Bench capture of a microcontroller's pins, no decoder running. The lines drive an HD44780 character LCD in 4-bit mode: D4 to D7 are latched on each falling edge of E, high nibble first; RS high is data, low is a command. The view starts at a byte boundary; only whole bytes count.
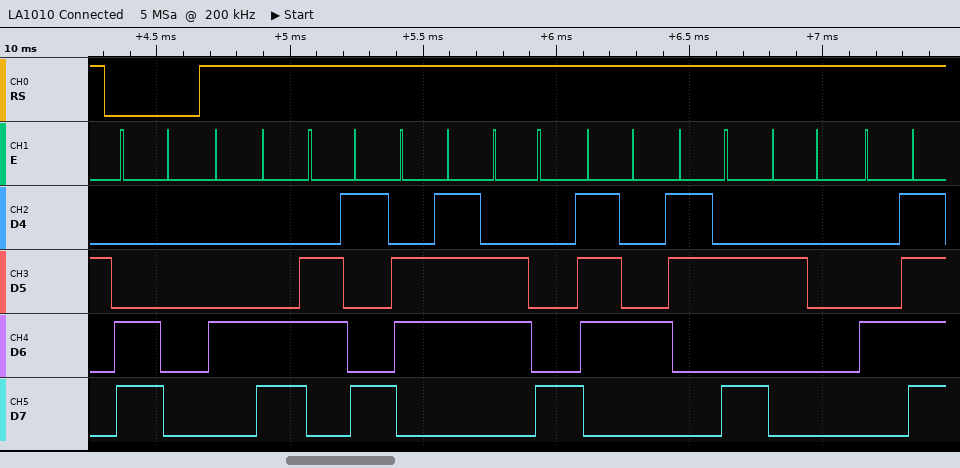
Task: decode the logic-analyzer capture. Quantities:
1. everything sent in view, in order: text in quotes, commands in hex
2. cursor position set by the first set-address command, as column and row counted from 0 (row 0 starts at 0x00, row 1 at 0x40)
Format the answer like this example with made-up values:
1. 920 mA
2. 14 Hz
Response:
1. 0xC0 "Light: O"
2. column 0, row 1
